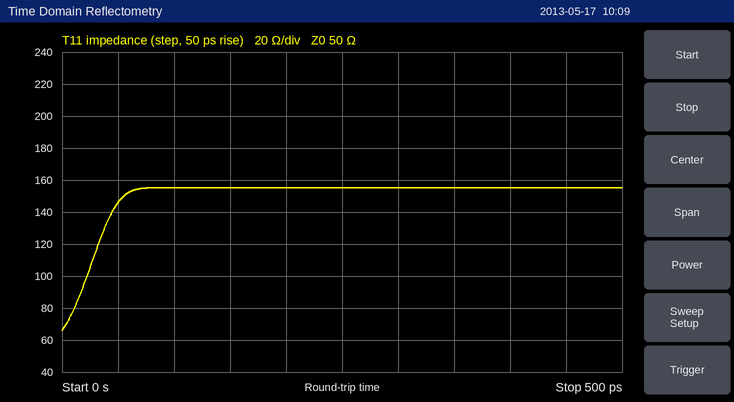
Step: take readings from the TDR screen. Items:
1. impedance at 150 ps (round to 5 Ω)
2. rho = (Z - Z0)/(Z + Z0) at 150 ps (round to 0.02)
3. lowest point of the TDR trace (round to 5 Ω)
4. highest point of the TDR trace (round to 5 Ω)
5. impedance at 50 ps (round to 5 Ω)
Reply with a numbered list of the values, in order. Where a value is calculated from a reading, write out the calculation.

1. 155 Ω
2. (155 − 50)/(155 + 50) ≈ +0.512, so +0.52 to the nearest 0.02
3. 65 Ω
4. 155 Ω
5. 145 Ω
